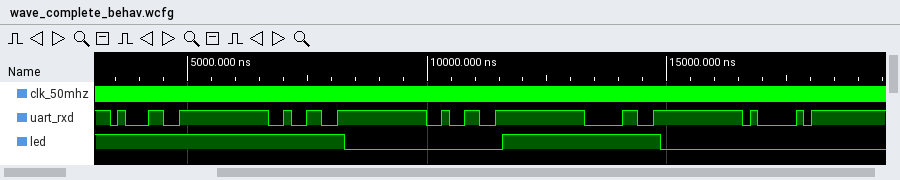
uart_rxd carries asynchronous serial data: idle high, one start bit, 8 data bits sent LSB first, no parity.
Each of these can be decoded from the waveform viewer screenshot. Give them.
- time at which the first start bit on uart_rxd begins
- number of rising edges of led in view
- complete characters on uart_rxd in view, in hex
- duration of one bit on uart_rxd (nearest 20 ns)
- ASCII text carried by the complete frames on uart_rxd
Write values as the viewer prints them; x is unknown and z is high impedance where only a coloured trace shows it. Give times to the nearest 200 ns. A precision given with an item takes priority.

3400 ns
1
31, 32, 32, 30, 41
160 ns
"1220A"
